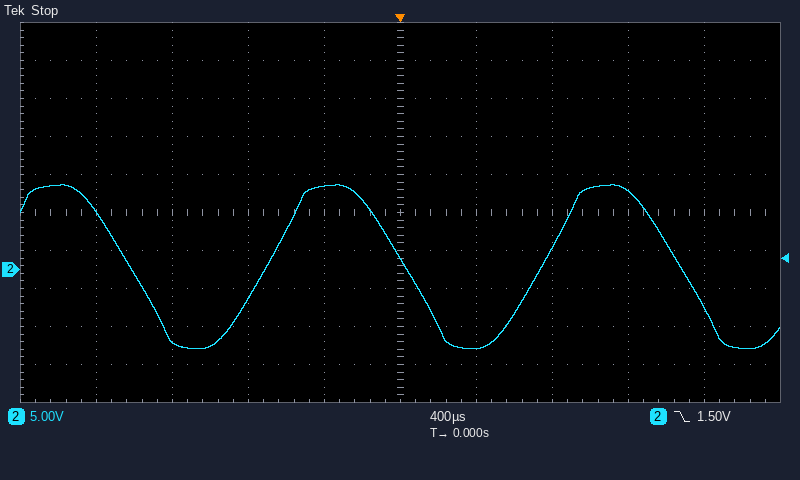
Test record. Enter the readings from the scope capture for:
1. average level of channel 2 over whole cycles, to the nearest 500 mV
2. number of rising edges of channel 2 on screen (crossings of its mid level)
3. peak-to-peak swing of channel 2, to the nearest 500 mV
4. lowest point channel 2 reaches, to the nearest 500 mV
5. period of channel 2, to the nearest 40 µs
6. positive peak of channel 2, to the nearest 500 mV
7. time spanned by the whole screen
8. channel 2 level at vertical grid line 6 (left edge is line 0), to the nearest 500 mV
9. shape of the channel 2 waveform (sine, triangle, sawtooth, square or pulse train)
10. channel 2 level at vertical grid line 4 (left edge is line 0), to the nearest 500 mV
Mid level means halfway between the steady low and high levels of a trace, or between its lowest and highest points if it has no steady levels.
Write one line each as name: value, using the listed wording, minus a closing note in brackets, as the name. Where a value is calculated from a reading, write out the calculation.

average level of channel 2 over whole cycles, to the nearest 500 mV: (11.0 V + (-10.5 V)) / 2 ≈ 250 mV, so 500 mV to the nearest 500 mV
number of rising edges of channel 2 on screen: 2
peak-to-peak swing of channel 2, to the nearest 500 mV: 11.0 V − (-10.5 V) = 21.5 V
lowest point channel 2 reaches, to the nearest 500 mV: -10.5 V
period of channel 2, to the nearest 40 µs: 1.44 ms
positive peak of channel 2, to the nearest 500 mV: 11.0 V
time spanned by the whole screen: 4 ms
channel 2 level at vertical grid line 6 (left edge is line 0), to the nearest 500 mV: -10.5 V
shape of the channel 2 waveform: sine
channel 2 level at vertical grid line 4 (left edge is line 0), to the nearest 500 mV: 11.0 V
